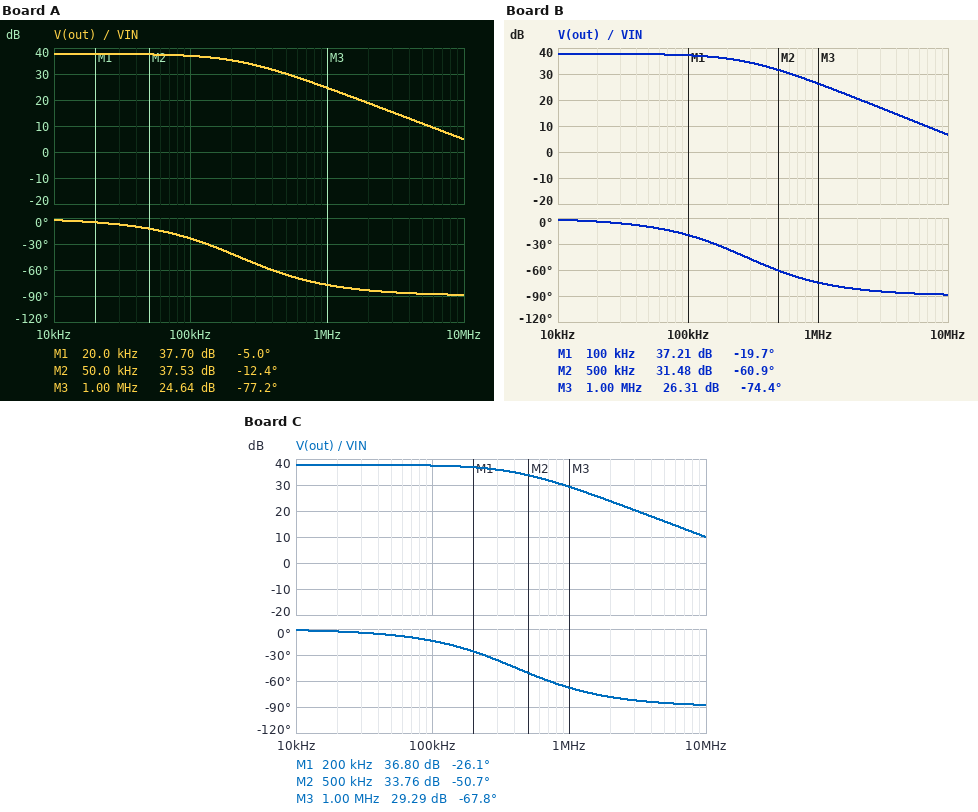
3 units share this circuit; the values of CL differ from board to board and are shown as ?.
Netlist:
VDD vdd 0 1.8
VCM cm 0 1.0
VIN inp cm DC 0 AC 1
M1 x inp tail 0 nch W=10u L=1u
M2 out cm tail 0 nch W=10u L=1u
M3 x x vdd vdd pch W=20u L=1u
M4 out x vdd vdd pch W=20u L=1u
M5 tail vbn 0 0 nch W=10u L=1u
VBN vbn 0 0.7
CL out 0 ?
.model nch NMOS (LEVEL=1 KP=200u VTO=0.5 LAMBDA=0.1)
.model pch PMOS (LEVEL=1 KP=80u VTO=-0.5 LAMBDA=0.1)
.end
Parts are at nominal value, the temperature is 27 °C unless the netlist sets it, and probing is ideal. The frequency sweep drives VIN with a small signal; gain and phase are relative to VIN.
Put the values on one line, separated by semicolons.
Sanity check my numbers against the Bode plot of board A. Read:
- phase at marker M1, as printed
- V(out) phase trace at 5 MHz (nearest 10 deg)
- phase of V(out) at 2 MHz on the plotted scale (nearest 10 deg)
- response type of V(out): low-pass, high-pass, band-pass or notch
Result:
-5.0 deg; -90 deg; -80 deg; low-pass
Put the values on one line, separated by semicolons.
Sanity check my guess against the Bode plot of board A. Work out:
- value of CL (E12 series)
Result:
2.7 pF
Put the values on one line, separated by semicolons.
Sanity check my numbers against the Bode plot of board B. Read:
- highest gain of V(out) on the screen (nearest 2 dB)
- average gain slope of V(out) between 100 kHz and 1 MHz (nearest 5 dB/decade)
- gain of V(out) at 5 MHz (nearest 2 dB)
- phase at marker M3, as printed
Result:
38 dB; -10 dB/decade; 12 dB; -74.4 deg
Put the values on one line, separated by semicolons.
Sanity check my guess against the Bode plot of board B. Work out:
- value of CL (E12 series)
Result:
2.2 pF
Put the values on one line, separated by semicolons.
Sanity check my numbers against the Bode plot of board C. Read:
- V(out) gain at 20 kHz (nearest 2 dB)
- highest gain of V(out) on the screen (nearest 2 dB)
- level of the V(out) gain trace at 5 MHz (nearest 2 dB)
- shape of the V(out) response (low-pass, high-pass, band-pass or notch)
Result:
38 dB; 38 dB; 16 dB; low-pass
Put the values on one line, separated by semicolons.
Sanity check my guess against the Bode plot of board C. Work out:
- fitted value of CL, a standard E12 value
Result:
1.5 pF
